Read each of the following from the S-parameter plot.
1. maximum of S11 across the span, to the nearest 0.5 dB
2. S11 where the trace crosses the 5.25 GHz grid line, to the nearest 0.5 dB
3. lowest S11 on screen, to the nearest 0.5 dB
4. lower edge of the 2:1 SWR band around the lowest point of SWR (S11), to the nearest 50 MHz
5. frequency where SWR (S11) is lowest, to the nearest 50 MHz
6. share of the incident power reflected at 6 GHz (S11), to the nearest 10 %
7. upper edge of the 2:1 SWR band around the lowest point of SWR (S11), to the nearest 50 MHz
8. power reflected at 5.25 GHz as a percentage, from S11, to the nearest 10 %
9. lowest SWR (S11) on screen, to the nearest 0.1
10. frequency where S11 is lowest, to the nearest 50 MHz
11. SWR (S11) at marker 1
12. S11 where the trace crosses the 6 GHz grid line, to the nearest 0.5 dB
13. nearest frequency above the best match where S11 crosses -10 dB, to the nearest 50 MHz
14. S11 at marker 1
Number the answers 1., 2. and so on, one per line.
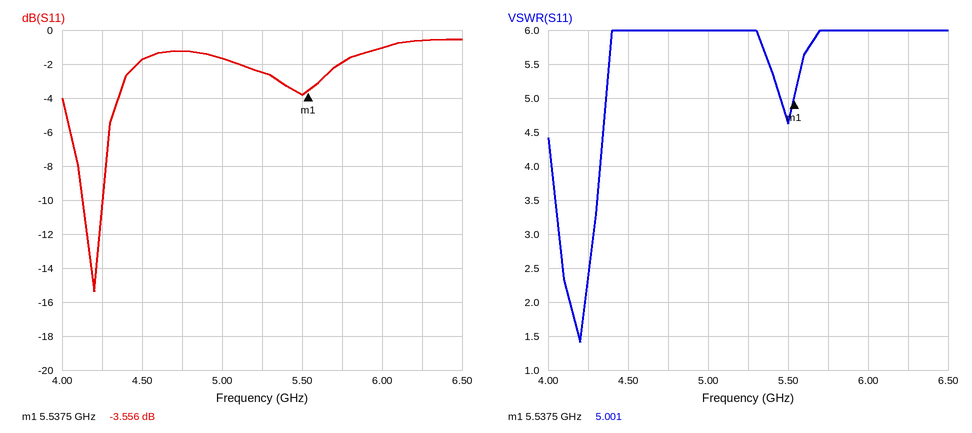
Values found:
1. -0.5 dB
2. -2.5 dB
3. -15.5 dB
4. 4.15 GHz
5. 4.20 GHz
6. 80 %
7. 4.25 GHz
8. 60 %
9. 1.4
10. 4.20 GHz
11. 5.001
12. -1.0 dB
13. 4.25 GHz
14. -3.556 dB
